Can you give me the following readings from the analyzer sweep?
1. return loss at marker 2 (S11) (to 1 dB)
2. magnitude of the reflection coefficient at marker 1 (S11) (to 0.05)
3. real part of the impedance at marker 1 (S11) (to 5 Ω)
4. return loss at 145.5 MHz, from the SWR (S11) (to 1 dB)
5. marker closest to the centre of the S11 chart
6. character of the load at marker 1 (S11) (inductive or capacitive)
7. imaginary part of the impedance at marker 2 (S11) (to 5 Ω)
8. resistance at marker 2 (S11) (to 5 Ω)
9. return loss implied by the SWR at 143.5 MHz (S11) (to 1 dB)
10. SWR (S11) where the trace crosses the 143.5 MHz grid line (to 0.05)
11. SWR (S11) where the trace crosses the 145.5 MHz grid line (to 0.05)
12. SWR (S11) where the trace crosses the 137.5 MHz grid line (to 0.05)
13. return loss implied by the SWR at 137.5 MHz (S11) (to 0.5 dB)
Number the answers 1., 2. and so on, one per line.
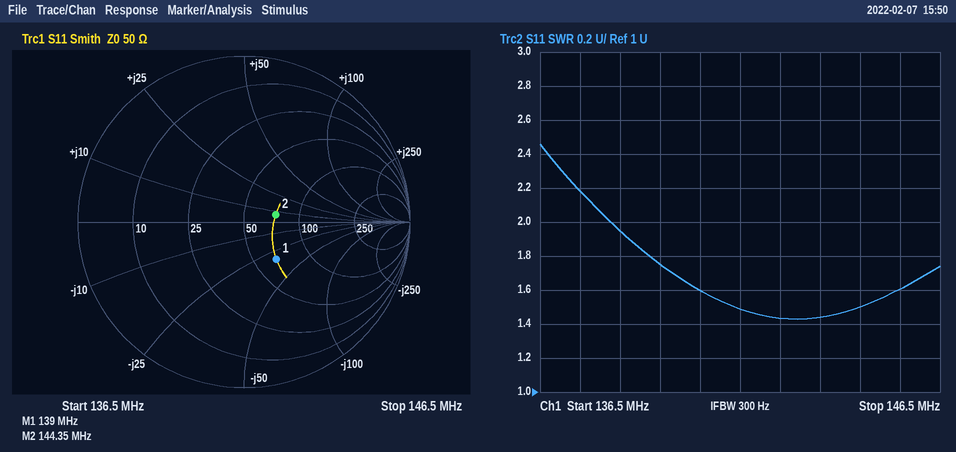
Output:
1. 14 dB
2. 0.30
3. 65 Ω
4. 13 dB
5. marker 2
6. capacitive
7. +5 Ω
8. 75 Ω
9. 15 dB
10. 1.45
11. 1.60
12. 2.20
13. 8.5 dB
